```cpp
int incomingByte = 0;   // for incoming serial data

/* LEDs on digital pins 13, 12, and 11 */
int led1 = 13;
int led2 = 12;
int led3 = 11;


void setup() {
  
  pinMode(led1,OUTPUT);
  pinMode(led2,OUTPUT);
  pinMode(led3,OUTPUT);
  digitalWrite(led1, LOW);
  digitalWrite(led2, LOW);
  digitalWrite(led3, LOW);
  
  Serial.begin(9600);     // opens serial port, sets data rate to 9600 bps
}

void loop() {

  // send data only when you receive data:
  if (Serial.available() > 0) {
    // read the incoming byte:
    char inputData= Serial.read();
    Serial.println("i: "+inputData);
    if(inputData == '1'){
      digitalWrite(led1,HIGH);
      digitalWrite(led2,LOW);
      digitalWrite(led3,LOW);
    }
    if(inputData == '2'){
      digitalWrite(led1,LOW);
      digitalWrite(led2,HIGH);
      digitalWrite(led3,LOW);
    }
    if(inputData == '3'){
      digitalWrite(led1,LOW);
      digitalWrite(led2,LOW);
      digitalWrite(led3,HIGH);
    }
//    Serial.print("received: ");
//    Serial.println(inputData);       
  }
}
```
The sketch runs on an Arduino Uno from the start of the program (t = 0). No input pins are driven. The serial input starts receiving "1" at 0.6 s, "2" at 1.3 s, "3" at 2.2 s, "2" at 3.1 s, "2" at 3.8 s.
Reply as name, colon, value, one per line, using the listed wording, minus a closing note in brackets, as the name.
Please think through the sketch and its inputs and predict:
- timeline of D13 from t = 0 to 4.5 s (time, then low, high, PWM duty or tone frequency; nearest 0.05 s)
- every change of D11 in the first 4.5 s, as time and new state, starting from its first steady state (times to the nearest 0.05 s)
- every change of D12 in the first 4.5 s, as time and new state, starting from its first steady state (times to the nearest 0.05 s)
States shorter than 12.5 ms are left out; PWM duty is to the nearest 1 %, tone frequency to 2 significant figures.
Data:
timeline of D13 from t = 0 to 4.5 s: 0 s low; 0.6 s high; 1.3 s low
every change of D11 in the first 4.5 s, as time and new state, starting from its first steady state: 0 s low; 2.2 s high; 3.1 s low
every change of D12 in the first 4.5 s, as time and new state, starting from its first steady state: 0 s low; 1.3 s high; 2.2 s low; 3.1 s high
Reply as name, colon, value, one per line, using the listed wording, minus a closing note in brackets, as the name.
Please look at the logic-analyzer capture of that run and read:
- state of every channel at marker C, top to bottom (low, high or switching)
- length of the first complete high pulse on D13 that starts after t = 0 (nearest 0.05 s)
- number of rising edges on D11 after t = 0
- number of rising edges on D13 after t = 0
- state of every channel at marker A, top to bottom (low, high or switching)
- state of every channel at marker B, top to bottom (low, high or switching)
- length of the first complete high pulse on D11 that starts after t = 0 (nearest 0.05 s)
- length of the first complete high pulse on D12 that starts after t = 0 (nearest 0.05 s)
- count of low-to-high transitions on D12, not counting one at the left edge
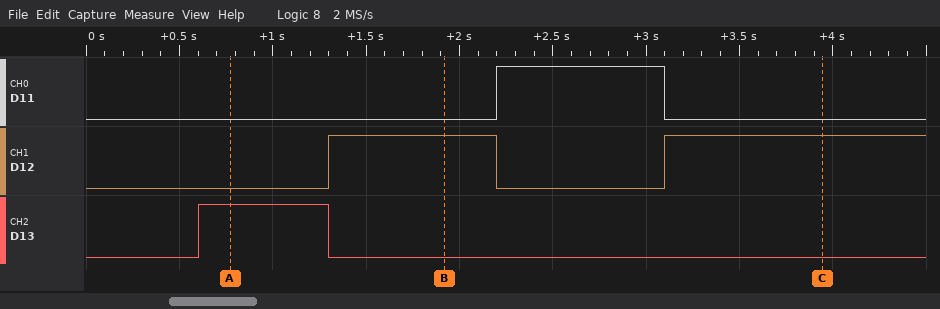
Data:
state of every channel at marker C, top to bottom: D11 low, D12 high, D13 low
length of the first complete high pulse on D13 that starts after t = 0: 0.70 s
number of rising edges on D11 after t = 0: 1
number of rising edges on D13 after t = 0: 1
state of every channel at marker A, top to bottom: D11 low, D12 low, D13 high
state of every channel at marker B, top to bottom: D11 low, D12 high, D13 low
length of the first complete high pulse on D11 that starts after t = 0: 0.90 s
length of the first complete high pulse on D12 that starts after t = 0: 0.90 s
count of low-to-high transitions on D12, not counting one at the left edge: 2
